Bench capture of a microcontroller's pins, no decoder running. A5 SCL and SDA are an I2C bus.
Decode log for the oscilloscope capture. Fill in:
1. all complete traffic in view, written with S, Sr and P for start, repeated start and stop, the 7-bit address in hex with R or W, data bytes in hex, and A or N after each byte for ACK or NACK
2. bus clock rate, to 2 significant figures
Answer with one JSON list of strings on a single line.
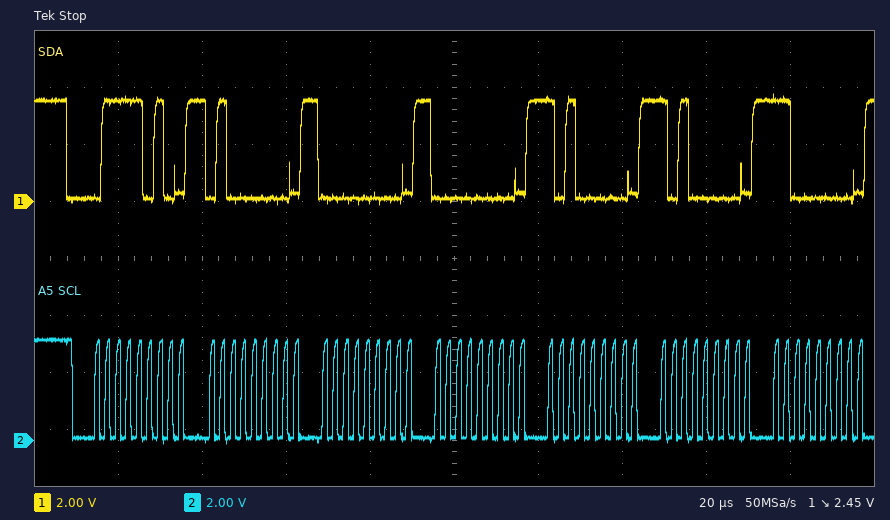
["S 3DW A 40 A 00 A 00 A A0 A A0 A C0 A", "400 kHz"]
